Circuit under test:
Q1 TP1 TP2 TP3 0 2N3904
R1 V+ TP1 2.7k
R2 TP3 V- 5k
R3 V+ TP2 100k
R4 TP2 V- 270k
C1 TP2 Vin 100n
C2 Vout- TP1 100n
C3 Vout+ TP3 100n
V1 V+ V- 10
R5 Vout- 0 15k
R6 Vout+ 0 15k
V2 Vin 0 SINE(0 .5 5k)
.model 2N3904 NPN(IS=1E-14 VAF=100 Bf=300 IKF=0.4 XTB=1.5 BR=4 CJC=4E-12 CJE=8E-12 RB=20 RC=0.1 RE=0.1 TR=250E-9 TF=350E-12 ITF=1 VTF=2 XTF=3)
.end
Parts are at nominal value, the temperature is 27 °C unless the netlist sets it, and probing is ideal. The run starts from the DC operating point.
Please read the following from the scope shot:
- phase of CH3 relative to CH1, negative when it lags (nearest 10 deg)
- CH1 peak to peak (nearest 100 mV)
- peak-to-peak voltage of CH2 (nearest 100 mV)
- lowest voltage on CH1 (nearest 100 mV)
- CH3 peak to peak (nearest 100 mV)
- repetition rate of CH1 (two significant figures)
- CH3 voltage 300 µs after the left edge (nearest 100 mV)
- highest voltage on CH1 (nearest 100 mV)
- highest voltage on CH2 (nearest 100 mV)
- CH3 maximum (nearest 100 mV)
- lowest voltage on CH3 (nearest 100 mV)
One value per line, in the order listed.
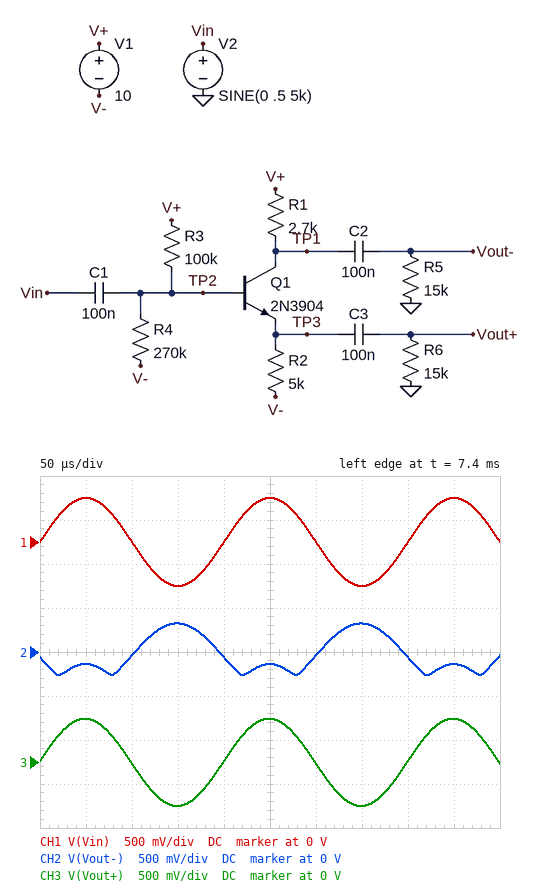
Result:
0 deg
1.0 V
600 mV
-500 mV
1.0 V
5.0 kHz
0 V
500 mV
300 mV
500 mV
-500 mV
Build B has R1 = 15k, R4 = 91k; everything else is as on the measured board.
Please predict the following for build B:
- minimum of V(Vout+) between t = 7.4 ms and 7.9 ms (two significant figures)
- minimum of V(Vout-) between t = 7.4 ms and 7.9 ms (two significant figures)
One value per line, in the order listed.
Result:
-490 mV
-270 mV
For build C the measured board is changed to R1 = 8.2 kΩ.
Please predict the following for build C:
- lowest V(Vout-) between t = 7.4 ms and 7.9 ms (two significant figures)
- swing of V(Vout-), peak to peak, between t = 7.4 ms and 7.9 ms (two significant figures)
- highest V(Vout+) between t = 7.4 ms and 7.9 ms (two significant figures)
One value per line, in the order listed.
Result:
-290 mV
630 mV
490 mV
